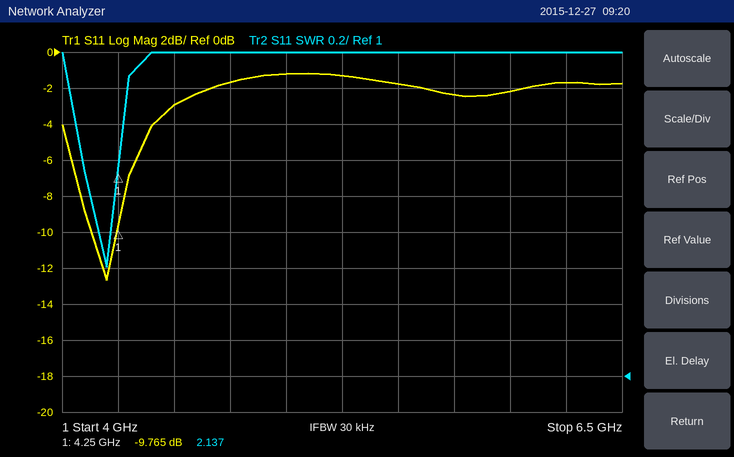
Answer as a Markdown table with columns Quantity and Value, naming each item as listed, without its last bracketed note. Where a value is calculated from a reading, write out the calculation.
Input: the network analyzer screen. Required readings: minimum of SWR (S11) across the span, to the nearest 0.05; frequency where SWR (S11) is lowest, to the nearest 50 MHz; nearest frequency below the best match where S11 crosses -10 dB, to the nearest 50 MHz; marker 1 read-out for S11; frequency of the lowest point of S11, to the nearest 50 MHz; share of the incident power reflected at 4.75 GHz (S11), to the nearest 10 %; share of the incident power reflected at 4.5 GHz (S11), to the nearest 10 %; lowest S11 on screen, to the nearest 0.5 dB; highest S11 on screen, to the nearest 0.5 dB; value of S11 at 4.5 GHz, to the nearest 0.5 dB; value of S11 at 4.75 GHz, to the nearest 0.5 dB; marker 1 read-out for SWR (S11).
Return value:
| Quantity | Value |
|---|---|
| minimum of SWR (S11) across the span, to the nearest 0.05 | 1.60 |
| frequency where SWR (S11) is lowest, to the nearest 50 MHz | 4.20 GHz |
| nearest frequency below the best match where S11 crosses -10 dB, to the nearest 50 MHz | 4.15 GHz |
| marker 1 read-out for S11 | -9.765 dB |
| frequency of the lowest point of S11, to the nearest 50 MHz | 4.20 GHz |
| share of the incident power reflected at 4.75 GHz (S11), to the nearest 10 % | 10^(-1.5/10) ≈ 70.8 %, so 70 % to the nearest 10 % |
| share of the incident power reflected at 4.5 GHz (S11), to the nearest 10 % | 10^(-3/10) ≈ 50 % |
| lowest S11 on screen, to the nearest 0.5 dB | -12.5 dB |
| highest S11 on screen, to the nearest 0.5 dB | -1.0 dB |
| value of S11 at 4.5 GHz, to the nearest 0.5 dB | -3.0 dB |
| value of S11 at 4.75 GHz, to the nearest 0.5 dB | -1.5 dB |
| marker 1 read-out for SWR | 2.137 |
